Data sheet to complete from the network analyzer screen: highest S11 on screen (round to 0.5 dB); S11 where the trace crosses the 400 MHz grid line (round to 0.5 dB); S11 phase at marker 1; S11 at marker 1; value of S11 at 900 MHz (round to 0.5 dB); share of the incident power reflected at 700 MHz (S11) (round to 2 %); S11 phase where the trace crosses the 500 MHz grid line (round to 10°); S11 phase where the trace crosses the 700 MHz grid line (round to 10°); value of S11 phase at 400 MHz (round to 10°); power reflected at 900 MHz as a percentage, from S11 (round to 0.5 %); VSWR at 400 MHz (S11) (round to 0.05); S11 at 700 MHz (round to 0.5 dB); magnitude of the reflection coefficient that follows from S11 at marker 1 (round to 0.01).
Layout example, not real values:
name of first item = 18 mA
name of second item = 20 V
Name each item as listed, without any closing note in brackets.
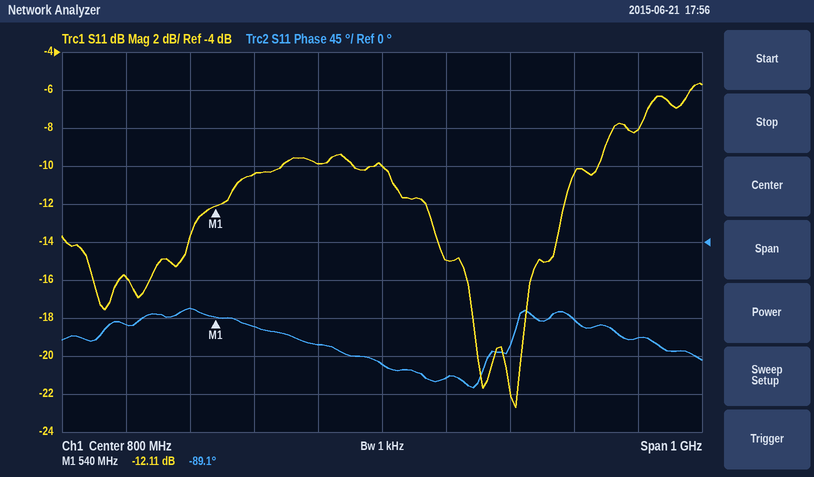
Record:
highest S11 on screen = -5.5 dB
S11 where the trace crosses the 400 MHz grid line = -16.0 dB
S11 phase at marker 1 = -89.1°
S11 at marker 1 = -12.11 dB
value of S11 at 900 MHz = -15.0 dB
share of the incident power reflected at 700 MHz (S11) = 10 %
S11 phase where the trace crosses the 500 MHz grid line = -80°
S11 phase where the trace crosses the 700 MHz grid line = -120°
value of S11 phase at 400 MHz = -100°
power reflected at 900 MHz as a percentage, from S11 = 3.0 %
VSWR at 400 MHz (S11) = 1.40
S11 at 700 MHz = -10.0 dB
magnitude of the reflection coefficient that follows from S11 at marker 1 = 0.25
